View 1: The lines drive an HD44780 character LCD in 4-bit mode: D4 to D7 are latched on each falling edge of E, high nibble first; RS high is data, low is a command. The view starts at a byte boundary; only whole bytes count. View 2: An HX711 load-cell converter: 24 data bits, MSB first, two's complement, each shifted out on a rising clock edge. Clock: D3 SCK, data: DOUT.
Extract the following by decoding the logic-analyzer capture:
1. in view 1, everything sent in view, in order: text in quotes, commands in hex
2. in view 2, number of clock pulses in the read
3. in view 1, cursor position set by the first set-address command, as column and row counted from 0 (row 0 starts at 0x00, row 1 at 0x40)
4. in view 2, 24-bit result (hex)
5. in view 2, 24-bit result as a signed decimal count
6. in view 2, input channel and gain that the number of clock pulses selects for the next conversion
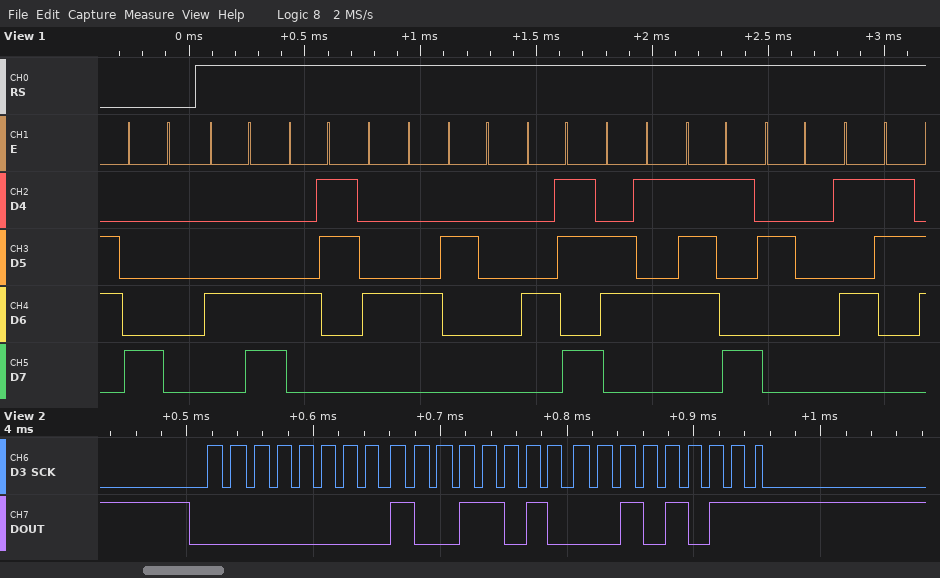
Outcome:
0x80 "LCD Key S"
25
column 0, row 0
0x009A2B
39467
channel A, gain 128
